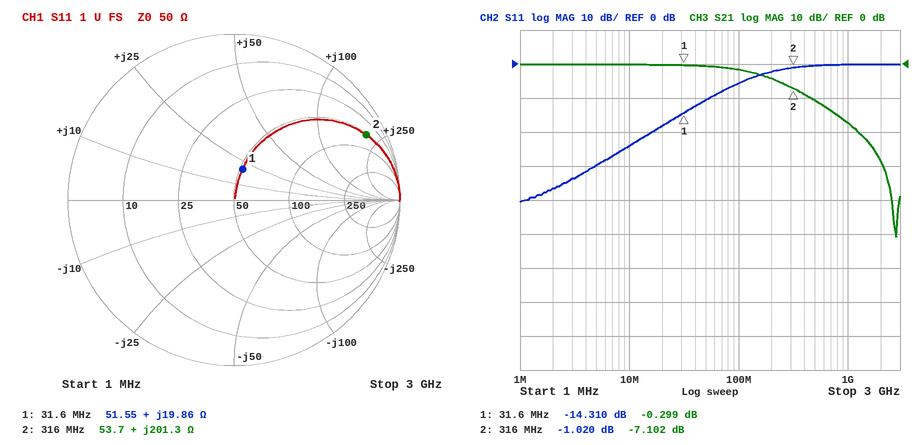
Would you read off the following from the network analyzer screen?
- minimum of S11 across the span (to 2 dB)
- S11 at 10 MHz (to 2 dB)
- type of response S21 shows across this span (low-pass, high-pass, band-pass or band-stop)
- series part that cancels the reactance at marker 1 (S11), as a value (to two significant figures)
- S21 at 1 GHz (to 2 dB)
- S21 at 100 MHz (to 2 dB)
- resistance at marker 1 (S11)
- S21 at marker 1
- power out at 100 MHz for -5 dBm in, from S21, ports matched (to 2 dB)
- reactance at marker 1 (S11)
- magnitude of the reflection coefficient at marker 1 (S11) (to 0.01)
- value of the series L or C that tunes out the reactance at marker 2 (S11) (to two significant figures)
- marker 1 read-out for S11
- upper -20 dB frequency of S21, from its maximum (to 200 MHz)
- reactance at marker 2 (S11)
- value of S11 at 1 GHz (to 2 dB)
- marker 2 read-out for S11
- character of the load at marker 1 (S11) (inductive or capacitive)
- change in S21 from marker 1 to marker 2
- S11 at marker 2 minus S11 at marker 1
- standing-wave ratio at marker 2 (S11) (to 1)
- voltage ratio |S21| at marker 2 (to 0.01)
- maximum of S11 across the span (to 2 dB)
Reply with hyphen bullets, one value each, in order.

- -40 dB
- -24 dB
- low-pass
- 250 pF
- -18 dB
- -2 dB
- 51.55 Ω
- -0.299 dB
- -6 dBm
- +19.86 Ω
- 0.19
- 2.5 pF
- -14.310 dB
- 1.2 GHz
- +201.3 Ω
- 0 dB
- -1.020 dB
- inductive
- -6.803 dB
- 13.290 dB
- 17
- 0.44
- 0 dB
